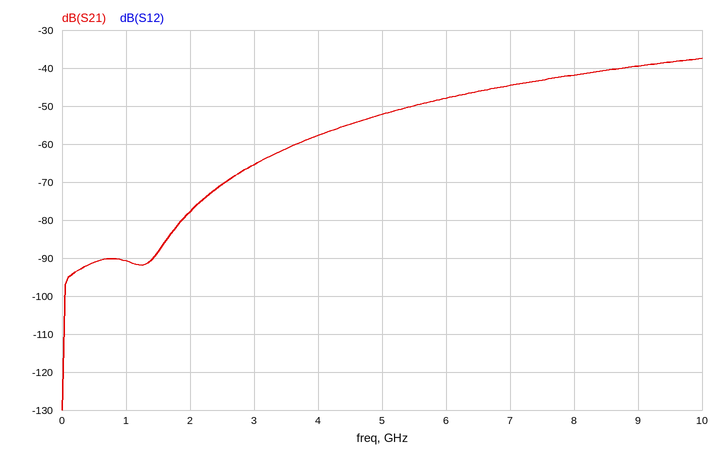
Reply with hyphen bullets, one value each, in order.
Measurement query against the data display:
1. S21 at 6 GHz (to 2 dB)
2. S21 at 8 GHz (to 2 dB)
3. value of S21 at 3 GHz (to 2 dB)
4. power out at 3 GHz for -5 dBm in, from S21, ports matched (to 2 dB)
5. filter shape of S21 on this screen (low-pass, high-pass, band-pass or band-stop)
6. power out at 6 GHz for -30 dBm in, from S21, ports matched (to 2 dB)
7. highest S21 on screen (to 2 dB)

- -48 dB
- -42 dB
- -66 dB
- -70 dBm
- high-pass
- -78 dBm
- -38 dB
